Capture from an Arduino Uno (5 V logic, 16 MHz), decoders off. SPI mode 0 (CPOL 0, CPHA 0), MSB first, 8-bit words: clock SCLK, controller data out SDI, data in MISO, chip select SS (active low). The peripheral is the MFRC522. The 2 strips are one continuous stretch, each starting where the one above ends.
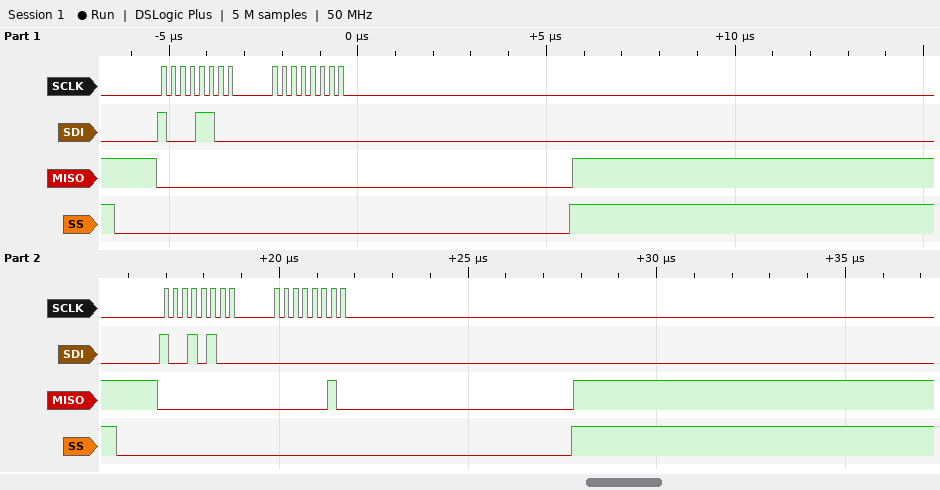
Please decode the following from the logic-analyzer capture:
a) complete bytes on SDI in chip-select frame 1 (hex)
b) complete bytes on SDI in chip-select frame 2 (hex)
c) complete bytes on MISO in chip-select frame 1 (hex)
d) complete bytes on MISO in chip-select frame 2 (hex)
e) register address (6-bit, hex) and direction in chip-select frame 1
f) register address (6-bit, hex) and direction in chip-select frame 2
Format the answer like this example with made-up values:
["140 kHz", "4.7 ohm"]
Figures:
["8C 00", "94 00", "00 00", "00 02", "0x06 read", "0x0A read"]
